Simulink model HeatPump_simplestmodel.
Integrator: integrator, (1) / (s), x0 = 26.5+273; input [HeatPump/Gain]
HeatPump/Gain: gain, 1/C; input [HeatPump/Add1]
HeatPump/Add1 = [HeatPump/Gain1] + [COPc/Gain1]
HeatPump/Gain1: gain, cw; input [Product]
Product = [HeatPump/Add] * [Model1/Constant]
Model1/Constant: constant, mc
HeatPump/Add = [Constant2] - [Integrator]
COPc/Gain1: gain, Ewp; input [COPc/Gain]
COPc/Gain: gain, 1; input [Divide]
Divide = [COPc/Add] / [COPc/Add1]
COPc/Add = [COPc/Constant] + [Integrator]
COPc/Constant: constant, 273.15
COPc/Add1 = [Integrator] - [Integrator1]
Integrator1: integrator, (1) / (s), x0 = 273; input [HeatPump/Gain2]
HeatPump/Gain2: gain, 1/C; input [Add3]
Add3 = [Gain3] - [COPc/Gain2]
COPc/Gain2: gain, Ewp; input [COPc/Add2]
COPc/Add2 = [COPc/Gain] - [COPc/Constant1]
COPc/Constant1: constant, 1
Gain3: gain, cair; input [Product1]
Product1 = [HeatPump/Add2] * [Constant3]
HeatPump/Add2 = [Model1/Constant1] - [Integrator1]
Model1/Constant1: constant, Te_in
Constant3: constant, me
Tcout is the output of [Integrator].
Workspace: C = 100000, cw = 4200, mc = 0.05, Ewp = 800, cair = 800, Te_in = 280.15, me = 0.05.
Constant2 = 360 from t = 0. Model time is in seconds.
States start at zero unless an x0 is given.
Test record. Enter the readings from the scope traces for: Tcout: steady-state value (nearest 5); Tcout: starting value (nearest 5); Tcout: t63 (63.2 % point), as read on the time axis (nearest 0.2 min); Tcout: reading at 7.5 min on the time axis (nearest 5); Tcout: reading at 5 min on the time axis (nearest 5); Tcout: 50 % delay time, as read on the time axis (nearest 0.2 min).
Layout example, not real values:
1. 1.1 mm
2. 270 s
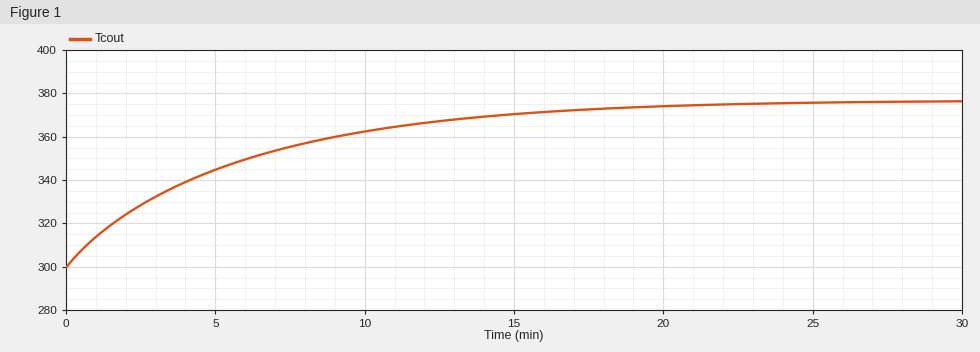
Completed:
1. 375
2. 300
3. 5.6 min
4. 355
5. 345
6. 3.8 min
